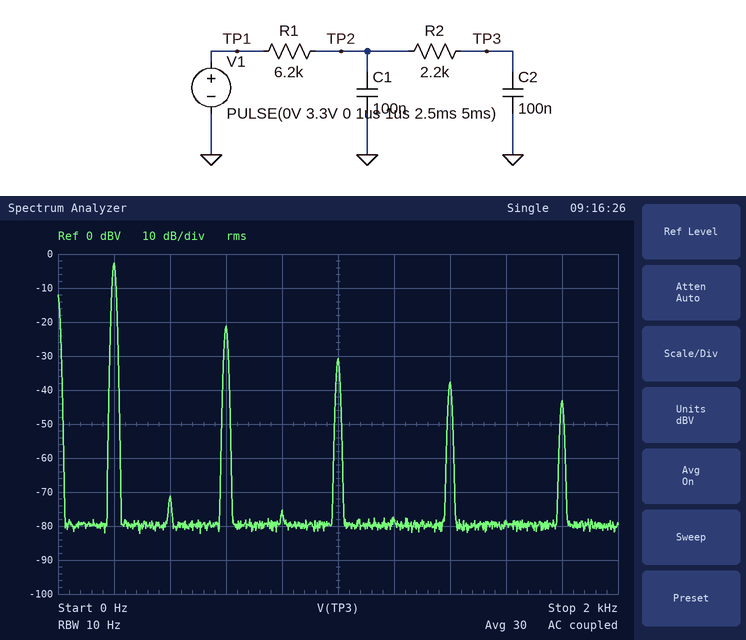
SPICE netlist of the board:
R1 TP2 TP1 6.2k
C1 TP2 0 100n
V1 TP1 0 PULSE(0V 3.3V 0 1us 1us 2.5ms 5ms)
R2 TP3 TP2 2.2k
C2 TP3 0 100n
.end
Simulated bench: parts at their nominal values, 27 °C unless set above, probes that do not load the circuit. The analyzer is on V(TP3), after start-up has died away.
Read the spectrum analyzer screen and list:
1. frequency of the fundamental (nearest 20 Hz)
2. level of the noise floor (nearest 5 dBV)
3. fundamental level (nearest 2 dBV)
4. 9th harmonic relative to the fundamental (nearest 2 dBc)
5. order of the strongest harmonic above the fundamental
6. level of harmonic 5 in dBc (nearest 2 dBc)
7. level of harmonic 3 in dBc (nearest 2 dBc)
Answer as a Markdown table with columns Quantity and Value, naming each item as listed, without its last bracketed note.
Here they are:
| Quantity | Value |
|---|---|
| frequency of the fundamental | 200 Hz |
| level of the noise floor | -80 dBV |
| fundamental level | -2 dBV |
| 9th harmonic relative to the fundamental | -40 dBc |
| order of the strongest harmonic above the fundamental | 3 |
| level of harmonic 5 in dBc | -28 dBc |
| level of harmonic 3 in dBc | -18 dBc |
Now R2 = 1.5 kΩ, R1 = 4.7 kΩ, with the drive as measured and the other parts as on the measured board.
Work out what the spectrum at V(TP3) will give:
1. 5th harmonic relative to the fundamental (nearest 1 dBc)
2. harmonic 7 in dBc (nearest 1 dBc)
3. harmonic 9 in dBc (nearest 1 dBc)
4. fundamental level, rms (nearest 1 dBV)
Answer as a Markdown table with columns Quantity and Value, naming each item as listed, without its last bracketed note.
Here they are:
| Quantity | Value |
|---|---|
| 5th harmonic relative to the fundamental | -27 dBc |
| harmonic 7 in dBc | -33 dBc |
| harmonic 9 in dBc | -38 dBc |
| fundamental level, rms | -1 dBV |
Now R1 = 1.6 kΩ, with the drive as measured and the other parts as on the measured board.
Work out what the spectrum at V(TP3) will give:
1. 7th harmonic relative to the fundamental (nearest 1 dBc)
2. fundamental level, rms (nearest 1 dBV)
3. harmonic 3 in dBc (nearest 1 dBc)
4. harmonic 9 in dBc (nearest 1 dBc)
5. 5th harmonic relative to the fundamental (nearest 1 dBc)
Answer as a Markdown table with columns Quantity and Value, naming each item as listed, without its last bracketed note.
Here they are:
| Quantity | Value |
|---|---|
| 7th harmonic relative to the fundamental | -30 dBc |
| fundamental level, rms | 2 dBV |
| harmonic 3 in dBc | -15 dBc |
| harmonic 9 in dBc | -35 dBc |
| 5th harmonic relative to the fundamental | -23 dBc |
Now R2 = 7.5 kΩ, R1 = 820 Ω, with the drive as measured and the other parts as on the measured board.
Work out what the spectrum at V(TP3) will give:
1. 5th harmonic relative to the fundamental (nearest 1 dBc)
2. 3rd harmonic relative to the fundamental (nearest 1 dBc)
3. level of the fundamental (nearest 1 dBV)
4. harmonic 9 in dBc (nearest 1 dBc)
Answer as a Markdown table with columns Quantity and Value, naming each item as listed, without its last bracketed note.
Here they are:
| Quantity | Value |
|---|---|
| 5th harmonic relative to the fundamental | -26 dBc |
| 3rd harmonic relative to the fundamental | -17 dBc |
| level of the fundamental | 0 dBV |
| harmonic 9 in dBc | -38 dBc |
